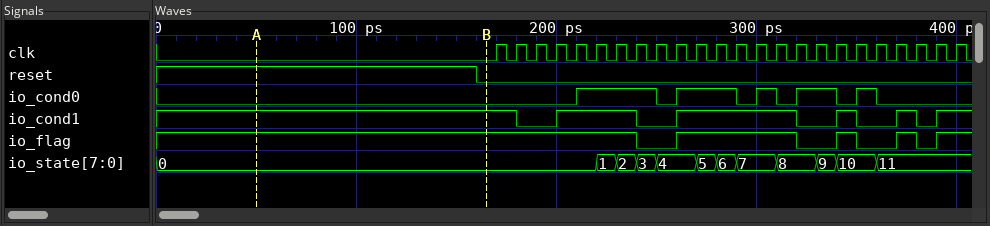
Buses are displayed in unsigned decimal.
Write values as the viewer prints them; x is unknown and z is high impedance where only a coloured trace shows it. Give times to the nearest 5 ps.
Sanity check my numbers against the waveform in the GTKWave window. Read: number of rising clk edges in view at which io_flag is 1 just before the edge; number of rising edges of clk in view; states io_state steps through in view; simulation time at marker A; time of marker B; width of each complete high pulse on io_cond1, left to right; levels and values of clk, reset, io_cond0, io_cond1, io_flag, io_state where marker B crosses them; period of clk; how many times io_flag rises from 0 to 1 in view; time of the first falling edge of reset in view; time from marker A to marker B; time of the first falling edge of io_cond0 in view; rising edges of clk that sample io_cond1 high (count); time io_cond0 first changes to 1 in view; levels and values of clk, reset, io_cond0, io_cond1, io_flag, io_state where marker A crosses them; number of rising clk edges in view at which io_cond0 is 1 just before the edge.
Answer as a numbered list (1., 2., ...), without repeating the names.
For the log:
1. 17
2. 24
3. 0, 1, 2, 3, 4, 5, 6, 7, 8, 9, 10, 11
4. 50 ps
5. 165 ps
6. 40 ps, 60 ps, 10 ps, 10 ps
7. clk=0, reset=0, io_cond0=0, io_cond1=1, io_flag=1, io_state=0
8. 10 ps
9. 4
10. 160 ps
11. 115 ps
12. 250 ps
13. 15
14. 210 ps
15. clk=0, reset=1, io_cond0=0, io_cond1=1, io_flag=1, io_state=0
16. 11
